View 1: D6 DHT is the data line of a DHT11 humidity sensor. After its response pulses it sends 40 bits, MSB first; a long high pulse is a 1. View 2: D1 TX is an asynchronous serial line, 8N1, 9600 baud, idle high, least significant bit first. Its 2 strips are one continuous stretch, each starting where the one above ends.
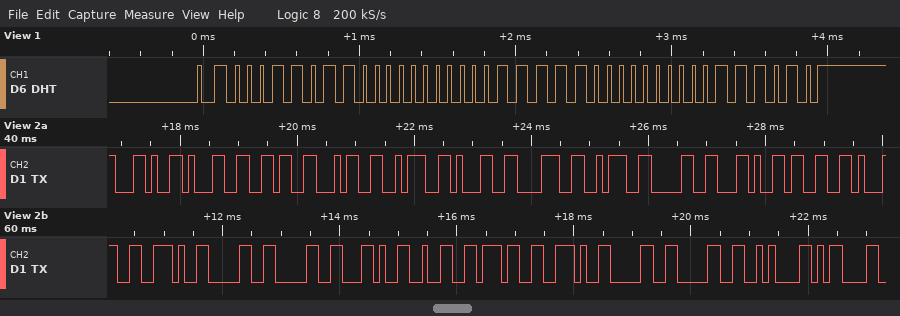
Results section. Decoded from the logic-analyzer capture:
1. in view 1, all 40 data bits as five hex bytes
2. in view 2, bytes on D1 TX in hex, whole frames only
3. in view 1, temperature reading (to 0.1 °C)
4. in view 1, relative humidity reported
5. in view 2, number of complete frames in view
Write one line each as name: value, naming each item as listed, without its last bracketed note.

in view 1, all 40 data bits as five hex bytes: 1B 00 1F 00 3A
in view 2, bytes on D1 TX in hex, whole frames only: 2C 31 36 34 3A 31 38 3A 30 2C 33 31 2E 30 30 2C 32 37 2E 30 30 0A 0D
in view 1, temperature reading: 31.0 °C
in view 1, relative humidity reported: 27 %
in view 2, number of complete frames in view: 23
